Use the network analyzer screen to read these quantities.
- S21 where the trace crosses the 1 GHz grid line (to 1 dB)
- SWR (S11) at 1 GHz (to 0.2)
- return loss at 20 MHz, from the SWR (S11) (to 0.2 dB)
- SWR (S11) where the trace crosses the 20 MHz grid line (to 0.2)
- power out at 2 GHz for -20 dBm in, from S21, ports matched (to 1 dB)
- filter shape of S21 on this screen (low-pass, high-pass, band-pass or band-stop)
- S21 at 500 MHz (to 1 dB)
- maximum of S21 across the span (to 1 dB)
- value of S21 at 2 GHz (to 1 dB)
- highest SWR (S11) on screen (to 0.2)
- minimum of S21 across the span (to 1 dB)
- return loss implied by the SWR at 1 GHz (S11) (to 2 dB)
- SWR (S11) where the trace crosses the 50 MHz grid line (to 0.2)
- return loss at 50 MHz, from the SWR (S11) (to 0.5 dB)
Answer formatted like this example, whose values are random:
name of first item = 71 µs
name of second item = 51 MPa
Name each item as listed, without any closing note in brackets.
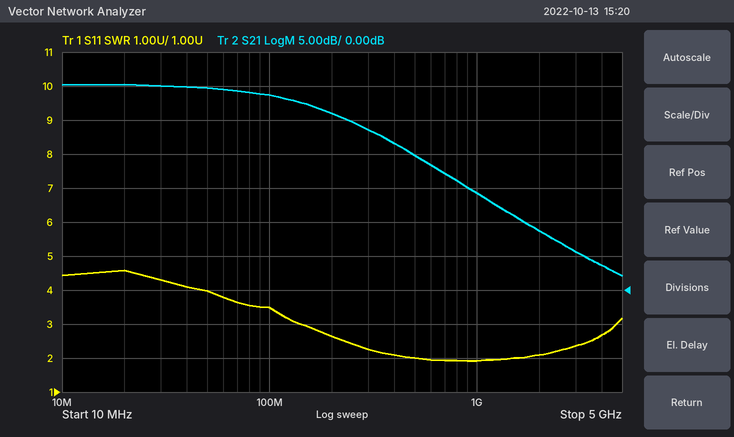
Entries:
S21 where the trace crosses the 1 GHz grid line = 14 dB
SWR (S11) at 1 GHz = 2.0
return loss at 20 MHz, from the SWR (S11) = 3.8 dB
SWR (S11) where the trace crosses the 20 MHz grid line = 4.6
power out at 2 GHz for -20 dBm in, from S21, ports matched = -11 dBm
filter shape of S21 on this screen = low-pass
S21 at 500 MHz = 20 dB
maximum of S21 across the span = 30 dB
value of S21 at 2 GHz = 9 dB
highest SWR (S11) on screen = 4.6
minimum of S21 across the span = 2 dB
return loss implied by the SWR at 1 GHz (S11) = 10 dB
SWR (S11) where the trace crosses the 50 MHz grid line = 4.0
return loss at 50 MHz, from the SWR (S11) = 4.5 dB
